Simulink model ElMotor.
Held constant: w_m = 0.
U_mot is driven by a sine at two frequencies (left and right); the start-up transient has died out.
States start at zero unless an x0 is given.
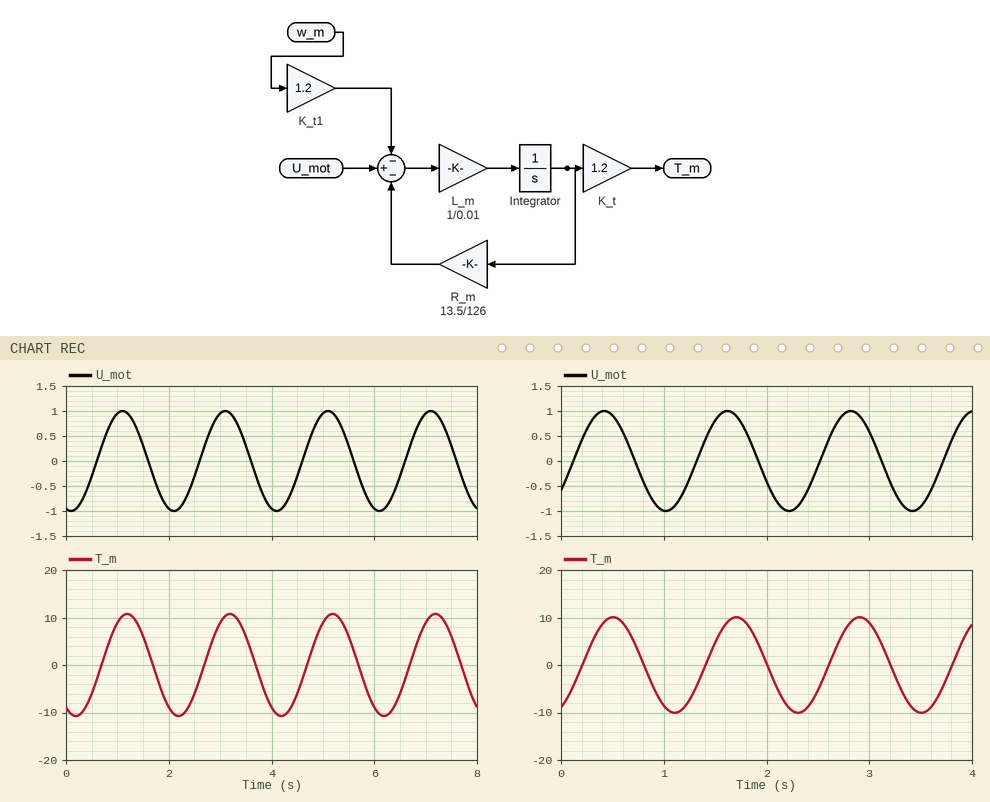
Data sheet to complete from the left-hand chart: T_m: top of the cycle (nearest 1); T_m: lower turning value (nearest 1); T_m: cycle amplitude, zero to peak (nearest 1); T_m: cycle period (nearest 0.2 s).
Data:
11
-11
11
2.0 s
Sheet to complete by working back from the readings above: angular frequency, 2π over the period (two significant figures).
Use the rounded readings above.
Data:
3.1 rad/s
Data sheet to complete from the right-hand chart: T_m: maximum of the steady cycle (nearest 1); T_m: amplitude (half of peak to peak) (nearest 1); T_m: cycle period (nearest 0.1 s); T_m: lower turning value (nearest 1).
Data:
10
10
1.2 s
-10
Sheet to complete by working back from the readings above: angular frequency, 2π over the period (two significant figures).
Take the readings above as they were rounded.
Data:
5.2 rad/s
